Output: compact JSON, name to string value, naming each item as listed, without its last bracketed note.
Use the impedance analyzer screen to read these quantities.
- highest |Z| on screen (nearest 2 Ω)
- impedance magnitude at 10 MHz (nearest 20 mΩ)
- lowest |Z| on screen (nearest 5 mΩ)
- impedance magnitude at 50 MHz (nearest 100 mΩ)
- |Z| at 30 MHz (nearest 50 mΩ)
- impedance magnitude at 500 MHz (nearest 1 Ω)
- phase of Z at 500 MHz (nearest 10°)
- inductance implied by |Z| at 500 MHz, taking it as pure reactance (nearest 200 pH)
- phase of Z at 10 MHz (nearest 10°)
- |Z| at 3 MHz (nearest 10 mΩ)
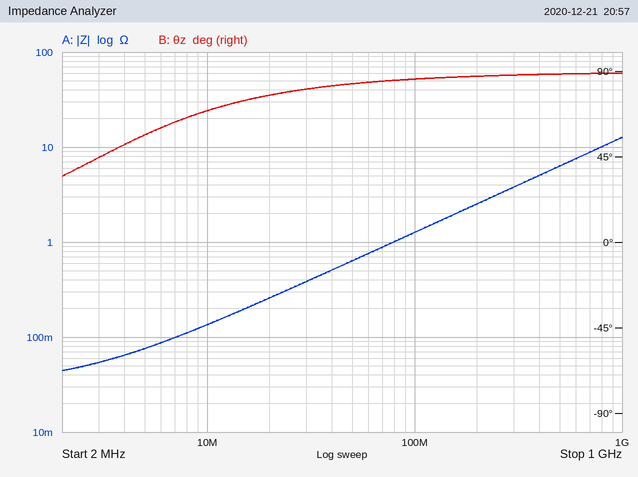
{"highest |Z| on screen": "12 Ω", "impedance magnitude at 10 MHz": "140 mΩ", "lowest |Z| on screen": "45 mΩ", "impedance magnitude at 50 MHz": "600 mΩ", "|Z| at 30 MHz": "400 mΩ", "impedance magnitude at 500 MHz": "6 Ω", "phase of Z at 500 MHz": "90°", "inductance implied by |Z| at 500 MHz, taking it as pure reactance": "2.0 nH", "phase of Z at 10 MHz": "70°", "|Z| at 3 MHz": "50 mΩ"}
